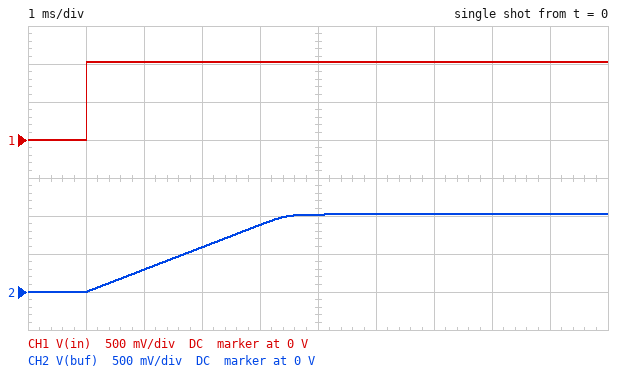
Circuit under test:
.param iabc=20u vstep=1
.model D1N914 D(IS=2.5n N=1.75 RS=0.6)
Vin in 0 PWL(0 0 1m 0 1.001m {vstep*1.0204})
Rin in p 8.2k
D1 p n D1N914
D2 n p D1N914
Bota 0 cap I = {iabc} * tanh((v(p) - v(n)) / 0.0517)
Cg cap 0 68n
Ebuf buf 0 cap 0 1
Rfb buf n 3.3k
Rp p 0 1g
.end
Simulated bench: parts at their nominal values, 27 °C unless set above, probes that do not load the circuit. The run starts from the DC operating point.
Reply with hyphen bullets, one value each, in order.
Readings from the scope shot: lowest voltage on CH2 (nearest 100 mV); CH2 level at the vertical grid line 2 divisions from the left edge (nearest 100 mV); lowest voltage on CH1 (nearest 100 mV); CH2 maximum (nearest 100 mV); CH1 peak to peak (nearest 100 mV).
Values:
- 0 V
- 300 mV
- 0 V
- 1.0 V
- 1.0 V
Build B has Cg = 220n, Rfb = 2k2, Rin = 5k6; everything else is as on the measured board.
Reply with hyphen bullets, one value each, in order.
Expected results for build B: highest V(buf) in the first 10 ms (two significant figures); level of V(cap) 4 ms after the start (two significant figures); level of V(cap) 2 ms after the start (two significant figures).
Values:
- 820 mV
- 270 mV
- 91 mV
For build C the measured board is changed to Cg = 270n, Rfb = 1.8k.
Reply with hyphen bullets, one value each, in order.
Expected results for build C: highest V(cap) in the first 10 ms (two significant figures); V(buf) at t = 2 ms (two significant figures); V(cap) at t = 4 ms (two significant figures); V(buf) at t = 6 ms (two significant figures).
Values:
- 670 mV
- 74 mV
- 220 mV
- 370 mV
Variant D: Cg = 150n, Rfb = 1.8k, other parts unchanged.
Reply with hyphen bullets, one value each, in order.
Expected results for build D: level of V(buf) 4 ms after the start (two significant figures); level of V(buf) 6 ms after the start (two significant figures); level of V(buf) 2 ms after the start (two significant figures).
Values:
- 400 mV
- 670 mV
- 130 mV
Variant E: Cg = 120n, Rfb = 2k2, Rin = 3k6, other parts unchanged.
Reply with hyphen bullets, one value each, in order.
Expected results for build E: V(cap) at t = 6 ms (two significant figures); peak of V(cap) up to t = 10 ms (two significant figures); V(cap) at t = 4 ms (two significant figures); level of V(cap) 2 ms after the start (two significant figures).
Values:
- 830 mV
- 1.0 V
- 500 mV
- 170 mV
